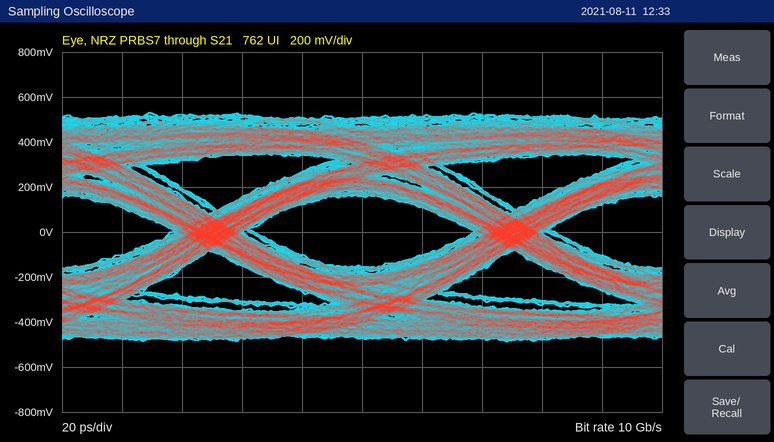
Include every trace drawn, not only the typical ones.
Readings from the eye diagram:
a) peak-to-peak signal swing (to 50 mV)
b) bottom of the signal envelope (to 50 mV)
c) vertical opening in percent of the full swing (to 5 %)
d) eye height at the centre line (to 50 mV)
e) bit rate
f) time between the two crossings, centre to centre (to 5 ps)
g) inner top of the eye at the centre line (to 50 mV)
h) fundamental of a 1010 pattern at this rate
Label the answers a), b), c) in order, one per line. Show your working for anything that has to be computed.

a) 1.00 V
b) -500 mV
c) 300 mV / 1.00 V ≈ 30 %
d) 300 mV
e) 10 Gb/s
f) 100 ps
g) 150 mV
h) 5 GHz
